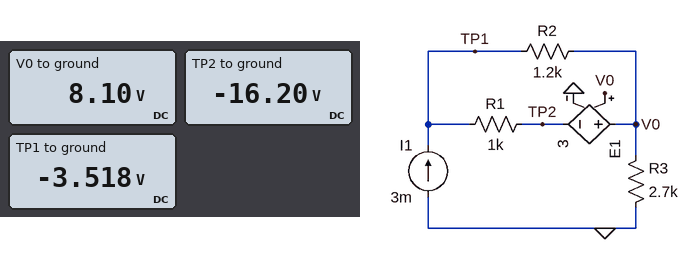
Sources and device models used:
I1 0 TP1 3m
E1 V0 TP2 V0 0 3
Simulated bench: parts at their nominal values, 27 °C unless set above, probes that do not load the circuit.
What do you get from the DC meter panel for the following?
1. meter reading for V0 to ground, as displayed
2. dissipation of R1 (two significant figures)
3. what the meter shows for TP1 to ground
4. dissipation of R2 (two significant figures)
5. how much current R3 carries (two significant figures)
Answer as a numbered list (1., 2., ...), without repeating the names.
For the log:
1. 8.10 V
2. 160 mW
3. -3.518 V
4. 110 mW
5. 3.0 mA
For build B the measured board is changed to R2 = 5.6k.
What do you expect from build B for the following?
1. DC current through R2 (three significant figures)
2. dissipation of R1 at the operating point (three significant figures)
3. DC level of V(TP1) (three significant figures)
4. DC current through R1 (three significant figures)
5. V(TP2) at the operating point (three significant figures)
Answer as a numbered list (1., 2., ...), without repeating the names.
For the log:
1. 3.23 mA
2. 38.8 mW
3. -9.97 V
4. 6.23 mA
5. -16.2 V
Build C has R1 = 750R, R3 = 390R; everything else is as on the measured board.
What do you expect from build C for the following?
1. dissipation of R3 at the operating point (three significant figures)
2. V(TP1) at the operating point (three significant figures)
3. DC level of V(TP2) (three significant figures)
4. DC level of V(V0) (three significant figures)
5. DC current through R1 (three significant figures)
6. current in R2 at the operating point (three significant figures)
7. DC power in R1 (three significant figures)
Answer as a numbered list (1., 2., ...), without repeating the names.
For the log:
1. 3.51 mW
2. 395 mV
3. -2.34 V
4. 1.17 V
5. 3.65 mA
6. 646 µA
7. 9.97 mW
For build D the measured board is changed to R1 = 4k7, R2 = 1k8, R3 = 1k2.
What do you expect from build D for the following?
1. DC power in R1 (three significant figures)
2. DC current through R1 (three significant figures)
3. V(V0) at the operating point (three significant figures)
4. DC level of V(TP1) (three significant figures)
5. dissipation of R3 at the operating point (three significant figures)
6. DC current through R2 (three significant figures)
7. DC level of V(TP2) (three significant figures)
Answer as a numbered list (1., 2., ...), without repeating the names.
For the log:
1. 29.2 mW
2. 2.49 mA
3. 3.60 V
4. 4.51 V
5. 10.8 mW
6. 508 µA
7. -7.20 V
